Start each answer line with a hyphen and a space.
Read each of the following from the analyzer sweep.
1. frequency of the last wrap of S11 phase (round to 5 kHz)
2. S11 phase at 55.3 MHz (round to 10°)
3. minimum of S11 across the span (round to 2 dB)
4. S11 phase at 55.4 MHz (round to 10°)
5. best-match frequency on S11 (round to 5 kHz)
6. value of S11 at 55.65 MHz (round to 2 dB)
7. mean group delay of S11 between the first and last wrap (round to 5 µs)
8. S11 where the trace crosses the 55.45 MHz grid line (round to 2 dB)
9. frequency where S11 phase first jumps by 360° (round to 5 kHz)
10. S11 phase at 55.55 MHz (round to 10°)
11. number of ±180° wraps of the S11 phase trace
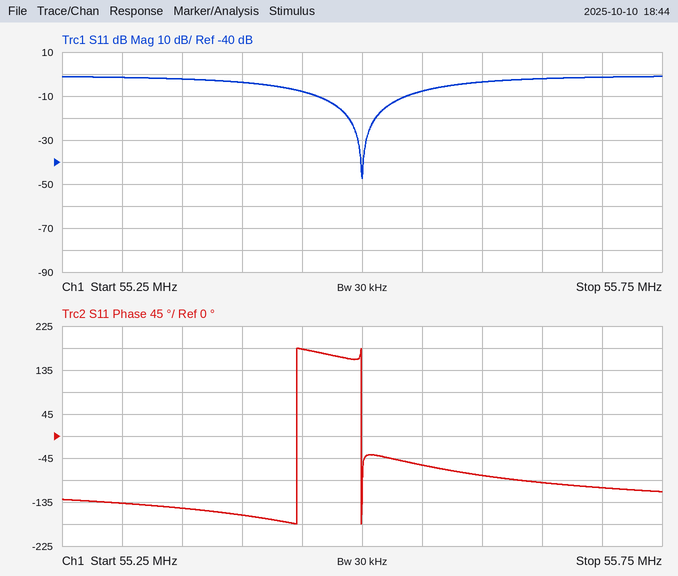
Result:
- 55.500 MHz
- -140°
- -48 dB
- -160°
- 55.500 MHz
- -2 dB
- 20 µs
- -8 dB
- 55.445 MHz
- -60°
- 2
